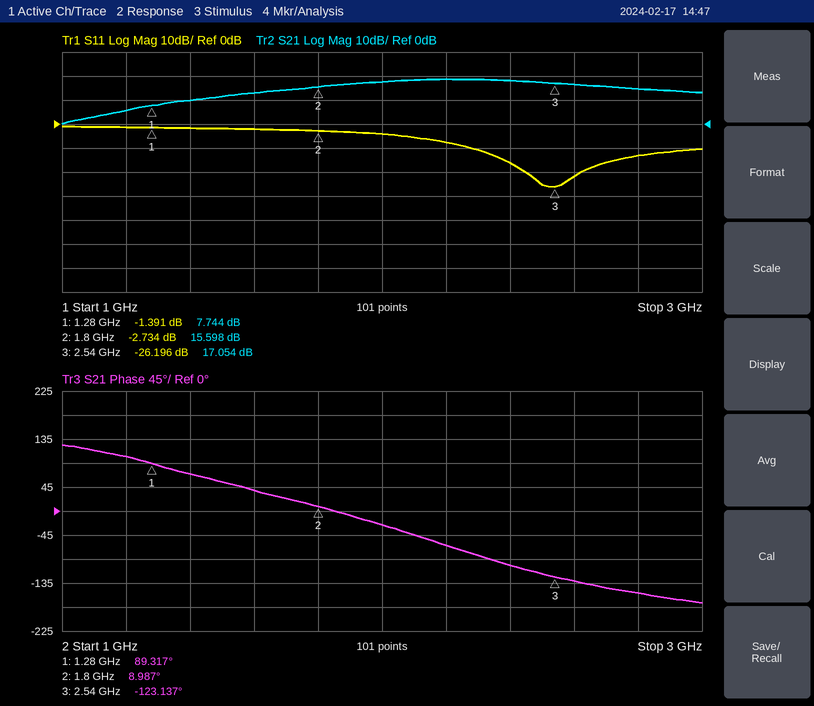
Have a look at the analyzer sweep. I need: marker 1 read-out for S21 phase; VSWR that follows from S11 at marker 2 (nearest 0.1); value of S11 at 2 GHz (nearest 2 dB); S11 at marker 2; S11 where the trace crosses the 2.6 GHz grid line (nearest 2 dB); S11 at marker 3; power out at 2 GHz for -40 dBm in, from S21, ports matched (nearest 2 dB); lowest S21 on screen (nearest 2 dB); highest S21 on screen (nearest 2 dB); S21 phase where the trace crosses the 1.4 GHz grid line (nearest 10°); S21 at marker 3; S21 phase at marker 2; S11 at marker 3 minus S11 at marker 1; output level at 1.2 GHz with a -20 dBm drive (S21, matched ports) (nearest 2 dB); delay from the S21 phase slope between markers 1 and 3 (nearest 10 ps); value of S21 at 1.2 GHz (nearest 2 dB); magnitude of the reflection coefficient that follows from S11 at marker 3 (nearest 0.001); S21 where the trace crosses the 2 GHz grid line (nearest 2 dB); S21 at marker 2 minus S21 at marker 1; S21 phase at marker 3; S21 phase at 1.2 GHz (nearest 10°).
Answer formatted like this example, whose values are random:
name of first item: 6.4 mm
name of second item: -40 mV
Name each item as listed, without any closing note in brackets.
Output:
marker 1 read-out for S21 phase: 89.317°
VSWR that follows from S11 at marker 2: 6.4
value of S11 at 2 GHz: -4 dB
S11 at marker 2: -2.734 dB
S11 where the trace crosses the 2.6 GHz grid line: -22 dB
S11 at marker 3: -26.196 dB
power out at 2 GHz for -40 dBm in, from S21, ports matched: -22 dBm
lowest S21 on screen: 0 dB
highest S21 on screen: 18 dB
S21 phase where the trace crosses the 1.4 GHz grid line: 70°
S21 at marker 3: 17.054 dB
S21 phase at marker 2: 8.987°
S11 at marker 3 minus S11 at marker 1: -24.805 dB
output level at 1.2 GHz with a -20 dBm drive (S21, matched ports): -14 dBm
delay from the S21 phase slope between markers 1 and 3: 470 ps
value of S21 at 1.2 GHz: 6 dB
magnitude of the reflection coefficient that follows from S11 at marker 3: 0.049
S21 where the trace crosses the 2 GHz grid line: 18 dB
S21 at marker 2 minus S21 at marker 1: 7.854 dB
S21 phase at marker 3: -123.137°
S21 phase at 1.2 GHz: 100°
